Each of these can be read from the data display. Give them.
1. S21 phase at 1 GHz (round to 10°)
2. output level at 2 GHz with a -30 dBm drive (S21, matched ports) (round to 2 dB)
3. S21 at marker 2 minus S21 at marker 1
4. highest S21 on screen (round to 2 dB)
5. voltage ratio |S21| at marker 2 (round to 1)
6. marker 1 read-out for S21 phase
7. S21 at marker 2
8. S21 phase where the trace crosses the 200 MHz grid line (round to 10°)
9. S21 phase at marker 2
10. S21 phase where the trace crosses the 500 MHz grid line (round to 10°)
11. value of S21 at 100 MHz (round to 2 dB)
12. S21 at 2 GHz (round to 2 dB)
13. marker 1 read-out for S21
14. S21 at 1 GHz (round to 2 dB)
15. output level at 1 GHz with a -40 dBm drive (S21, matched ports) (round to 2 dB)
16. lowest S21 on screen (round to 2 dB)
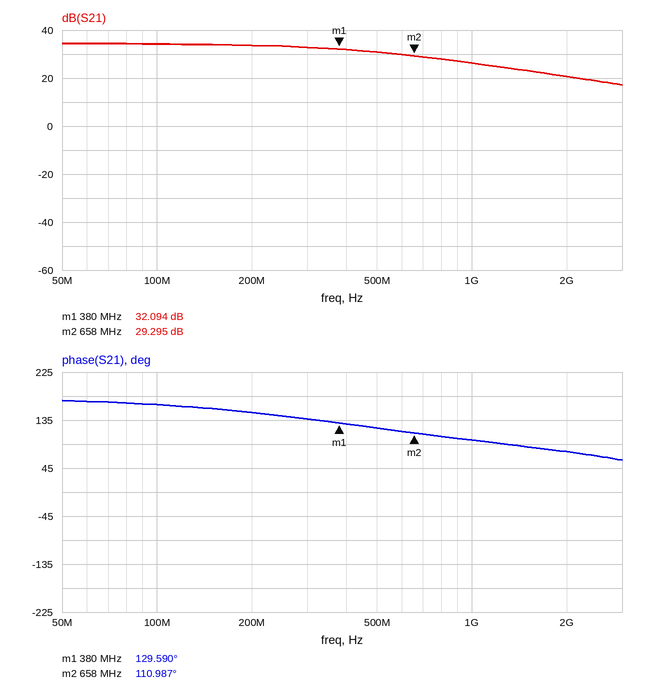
100°
-10 dBm
-2.799 dB
34 dB
29
129.590°
29.295 dB
150°
110.987°
120°
34 dB
20 dB
32.094 dB
26 dB
-14 dBm
18 dB
